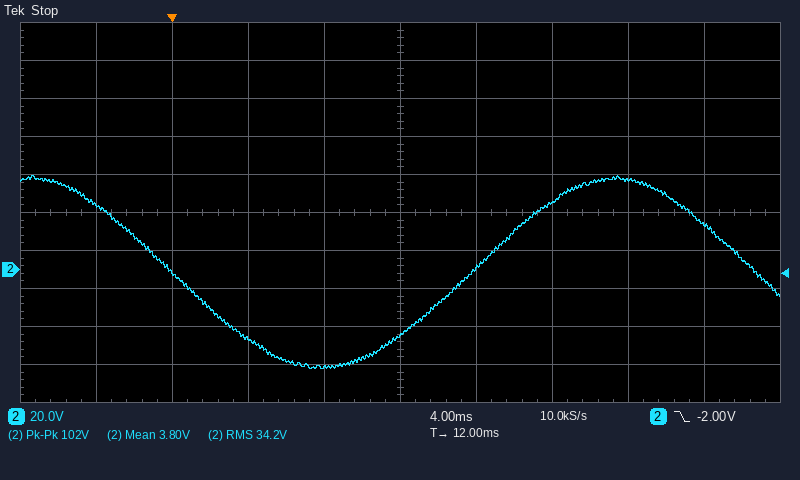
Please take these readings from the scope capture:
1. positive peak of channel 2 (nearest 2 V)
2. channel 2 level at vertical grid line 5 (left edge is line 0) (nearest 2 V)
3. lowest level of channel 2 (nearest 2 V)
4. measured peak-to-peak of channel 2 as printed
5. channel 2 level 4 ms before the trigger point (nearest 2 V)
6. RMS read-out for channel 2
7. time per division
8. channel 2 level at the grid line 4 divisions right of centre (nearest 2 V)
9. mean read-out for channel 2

50 V
-34 V
-52 V
102 V
34 V
34.2 V
4 ms
24 V
3.80 V
